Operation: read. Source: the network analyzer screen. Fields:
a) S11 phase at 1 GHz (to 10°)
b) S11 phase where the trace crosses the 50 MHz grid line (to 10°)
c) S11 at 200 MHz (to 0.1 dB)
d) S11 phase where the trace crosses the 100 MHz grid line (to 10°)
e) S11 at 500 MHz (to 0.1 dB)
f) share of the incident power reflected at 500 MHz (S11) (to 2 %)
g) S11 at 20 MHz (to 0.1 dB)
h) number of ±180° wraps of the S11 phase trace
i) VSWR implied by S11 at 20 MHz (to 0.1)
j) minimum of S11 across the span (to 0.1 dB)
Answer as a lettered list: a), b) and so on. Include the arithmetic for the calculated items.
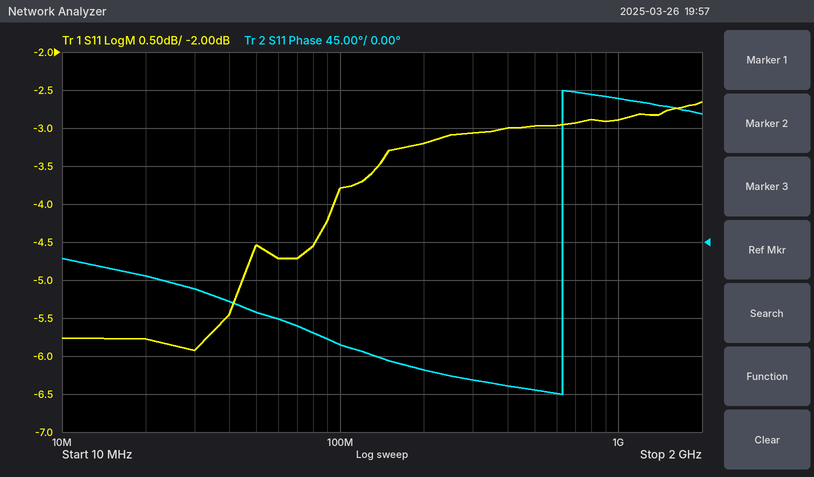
a) 170°
b) -80°
c) -3.2 dB
d) -120°
e) -3.0 dB
f) 10^(-3/10) ≈ 50 %
g) -5.8 dB
h) 1
i) |Γ| = 10^(-5.8/20) = 0.5129; VSWR = (1 + 0.5129)/(1 − 0.5129) ≈ 3.1
j) -5.9 dB
